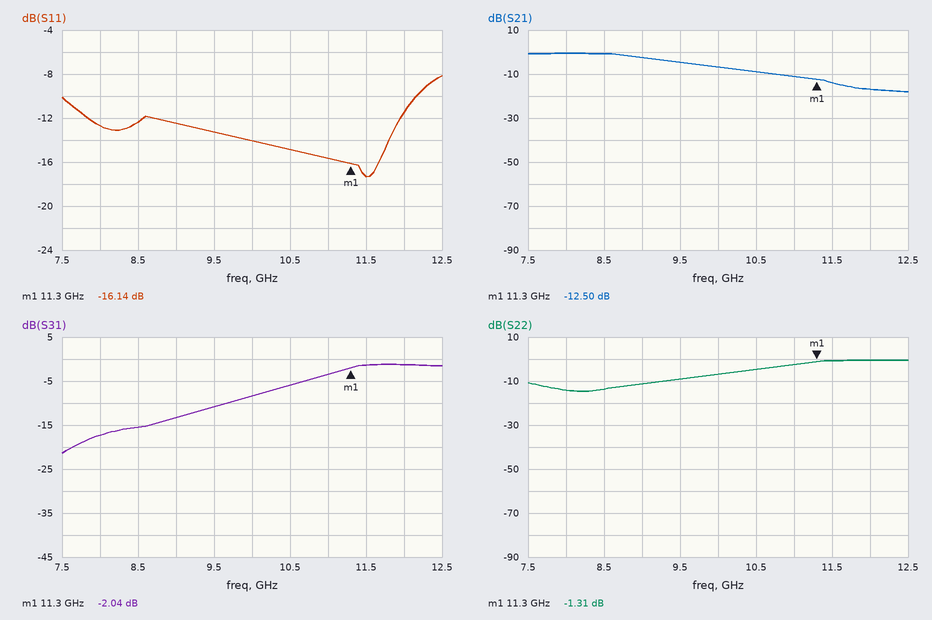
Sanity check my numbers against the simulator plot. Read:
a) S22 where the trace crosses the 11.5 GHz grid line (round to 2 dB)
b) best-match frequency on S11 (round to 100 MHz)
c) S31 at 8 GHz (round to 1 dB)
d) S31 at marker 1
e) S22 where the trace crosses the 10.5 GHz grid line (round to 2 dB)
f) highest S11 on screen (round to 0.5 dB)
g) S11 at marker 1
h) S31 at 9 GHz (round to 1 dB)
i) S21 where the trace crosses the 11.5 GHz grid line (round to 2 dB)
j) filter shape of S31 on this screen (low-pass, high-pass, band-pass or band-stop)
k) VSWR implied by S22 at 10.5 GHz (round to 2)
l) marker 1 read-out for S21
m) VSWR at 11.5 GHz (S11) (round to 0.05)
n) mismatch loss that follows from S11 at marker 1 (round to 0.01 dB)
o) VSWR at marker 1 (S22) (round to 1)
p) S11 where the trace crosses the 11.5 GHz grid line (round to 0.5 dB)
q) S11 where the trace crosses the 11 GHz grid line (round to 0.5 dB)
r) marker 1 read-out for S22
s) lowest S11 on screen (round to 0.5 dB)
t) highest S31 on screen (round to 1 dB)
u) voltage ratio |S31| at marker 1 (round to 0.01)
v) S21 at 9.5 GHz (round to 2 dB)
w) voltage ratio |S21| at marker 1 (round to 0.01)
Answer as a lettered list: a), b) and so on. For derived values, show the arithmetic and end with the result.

a) 0 dB
b) 11.5 GHz
c) -17 dB
d) -2.04 dB
e) -4 dB
f) -8.0 dB
g) -16.14 dB
h) -13 dB
i) -14 dB
j) high-pass
k) |Γ| = 10^(-4/20) = 0.6310; VSWR = (1 + 0.6310)/(1 − 0.6310) ≈ 4
l) -12.50 dB
m) |Γ| = 10^(-17.5/20) = 0.1334; VSWR = (1 + 0.1334)/(1 − 0.1334) ≈ 1.31, so 1.30 to the nearest 0.05
n) −10 log10(1 − 10^(-16.14/10)) ≈ 0.11 dB
o) (1 + 0.8600)/(1 − 0.8600) ≈ 13
p) -17.5 dB
q) -15.5 dB
r) -1.31 dB
s) -17.5 dB
t) -1 dB
u) 10^(-2.04/20) ≈ 0.79
v) -4 dB
w) 10^(-12.5/20) ≈ 0.24
